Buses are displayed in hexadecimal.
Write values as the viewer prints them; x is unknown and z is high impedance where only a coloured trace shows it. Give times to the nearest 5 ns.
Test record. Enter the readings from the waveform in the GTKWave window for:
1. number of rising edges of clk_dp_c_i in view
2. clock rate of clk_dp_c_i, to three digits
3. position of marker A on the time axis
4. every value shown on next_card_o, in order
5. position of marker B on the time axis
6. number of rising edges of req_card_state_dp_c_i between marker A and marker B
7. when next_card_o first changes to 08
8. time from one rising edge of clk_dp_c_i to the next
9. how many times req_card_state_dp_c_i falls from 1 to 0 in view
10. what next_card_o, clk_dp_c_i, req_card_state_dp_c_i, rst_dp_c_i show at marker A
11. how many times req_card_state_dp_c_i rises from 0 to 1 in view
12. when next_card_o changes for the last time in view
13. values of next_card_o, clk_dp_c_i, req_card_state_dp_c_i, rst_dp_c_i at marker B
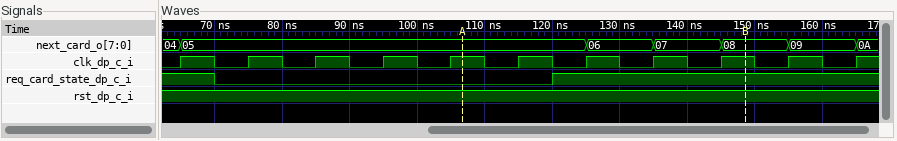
11
100 MHz
105 ns
04, 05, 06, 07, 08, 09, 0A
150 ns
1
145 ns
10 ns
1
next_card_o=05, clk_dp_c_i=1, req_card_state_dp_c_i=0, rst_dp_c_i=1
1
165 ns
next_card_o=08, clk_dp_c_i=1, req_card_state_dp_c_i=1, rst_dp_c_i=1
